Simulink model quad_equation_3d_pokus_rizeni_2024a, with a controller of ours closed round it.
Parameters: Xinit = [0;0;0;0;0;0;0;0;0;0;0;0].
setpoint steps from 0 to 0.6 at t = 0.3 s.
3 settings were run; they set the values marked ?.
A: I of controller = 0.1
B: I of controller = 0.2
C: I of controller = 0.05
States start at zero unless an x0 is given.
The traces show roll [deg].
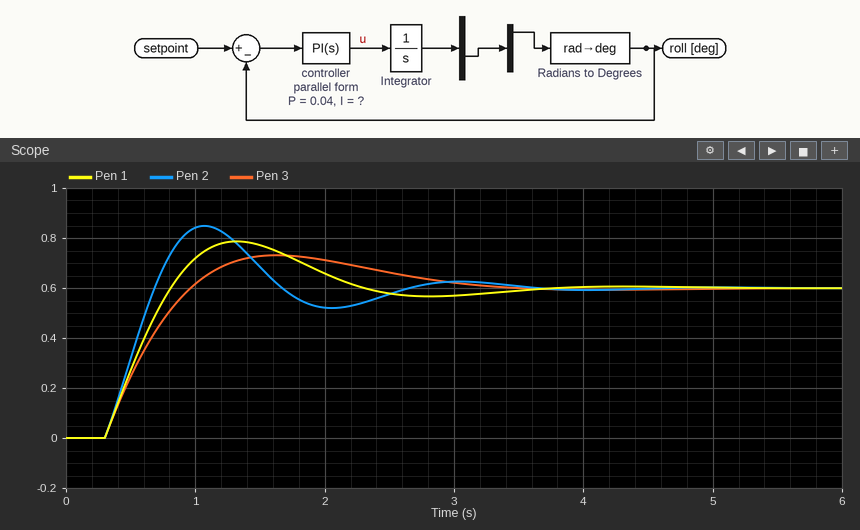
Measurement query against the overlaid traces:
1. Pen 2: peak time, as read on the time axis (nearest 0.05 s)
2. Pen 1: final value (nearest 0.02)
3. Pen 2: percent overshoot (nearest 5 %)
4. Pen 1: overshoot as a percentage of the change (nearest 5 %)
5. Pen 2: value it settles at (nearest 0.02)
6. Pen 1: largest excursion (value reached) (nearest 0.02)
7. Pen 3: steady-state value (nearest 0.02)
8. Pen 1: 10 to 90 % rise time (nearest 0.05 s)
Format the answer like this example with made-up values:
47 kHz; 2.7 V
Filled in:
1.05 s; 0.60; 40 %; 30 %; 0.60; 0.78; 0.60; 0.40 s
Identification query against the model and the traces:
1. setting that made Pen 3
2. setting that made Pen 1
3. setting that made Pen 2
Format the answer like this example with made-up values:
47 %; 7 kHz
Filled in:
C; A; B
